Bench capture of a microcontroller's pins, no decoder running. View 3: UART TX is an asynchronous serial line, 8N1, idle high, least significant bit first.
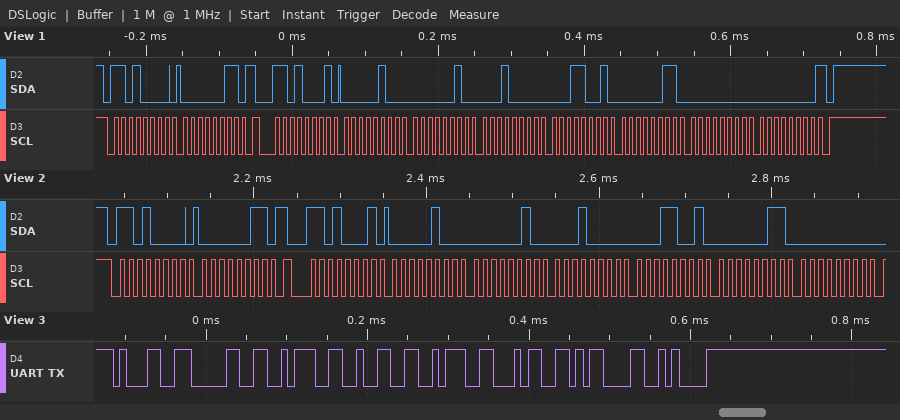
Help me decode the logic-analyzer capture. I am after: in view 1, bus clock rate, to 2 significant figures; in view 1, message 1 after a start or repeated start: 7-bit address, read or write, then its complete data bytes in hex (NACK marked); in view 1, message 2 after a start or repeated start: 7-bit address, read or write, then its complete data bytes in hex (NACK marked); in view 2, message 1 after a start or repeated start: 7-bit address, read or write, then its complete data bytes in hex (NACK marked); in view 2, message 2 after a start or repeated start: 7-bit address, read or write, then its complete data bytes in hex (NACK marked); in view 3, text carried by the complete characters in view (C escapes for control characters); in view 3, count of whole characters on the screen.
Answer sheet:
100 kHz
0x68 write: 03
0x68 read: 04 02 10 19 03 00 00 NACK
0x68 write: 03
0x68 read: 04 02 10 19 03 00
"10:2:4\r\n"
8
